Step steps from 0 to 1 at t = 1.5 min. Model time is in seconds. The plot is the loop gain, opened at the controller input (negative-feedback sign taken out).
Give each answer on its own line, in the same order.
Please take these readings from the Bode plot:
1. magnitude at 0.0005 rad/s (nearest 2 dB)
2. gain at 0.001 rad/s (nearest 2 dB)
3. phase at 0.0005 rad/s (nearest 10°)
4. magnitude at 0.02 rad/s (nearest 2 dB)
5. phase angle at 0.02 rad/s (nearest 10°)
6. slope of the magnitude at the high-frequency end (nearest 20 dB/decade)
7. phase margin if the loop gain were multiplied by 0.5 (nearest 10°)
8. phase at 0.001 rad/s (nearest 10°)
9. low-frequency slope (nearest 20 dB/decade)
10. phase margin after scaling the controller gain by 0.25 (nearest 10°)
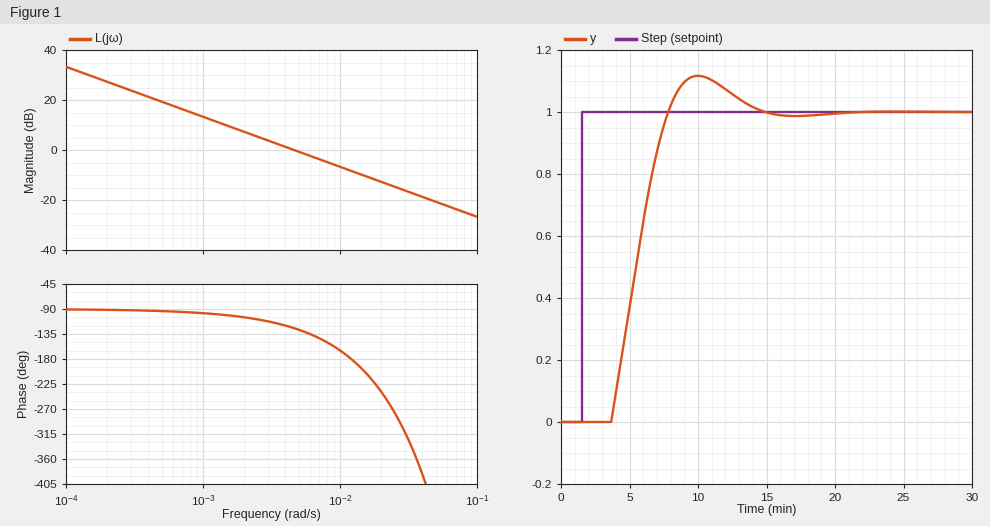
20 dB
14 dB
-90°
-12 dB
-240°
-20 dB/decade
70°
-100°
-20 dB/decade
80°
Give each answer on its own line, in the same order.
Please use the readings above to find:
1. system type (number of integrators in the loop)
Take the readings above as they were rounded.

1
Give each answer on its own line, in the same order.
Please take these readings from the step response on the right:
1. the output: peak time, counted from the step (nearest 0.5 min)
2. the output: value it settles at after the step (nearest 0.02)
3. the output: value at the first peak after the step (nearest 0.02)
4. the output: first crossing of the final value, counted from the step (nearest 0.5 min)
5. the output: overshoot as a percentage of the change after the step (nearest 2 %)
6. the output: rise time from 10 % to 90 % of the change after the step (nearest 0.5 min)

8.5 min
1.00
1.12
6.5 min
12 %
3.0 min
